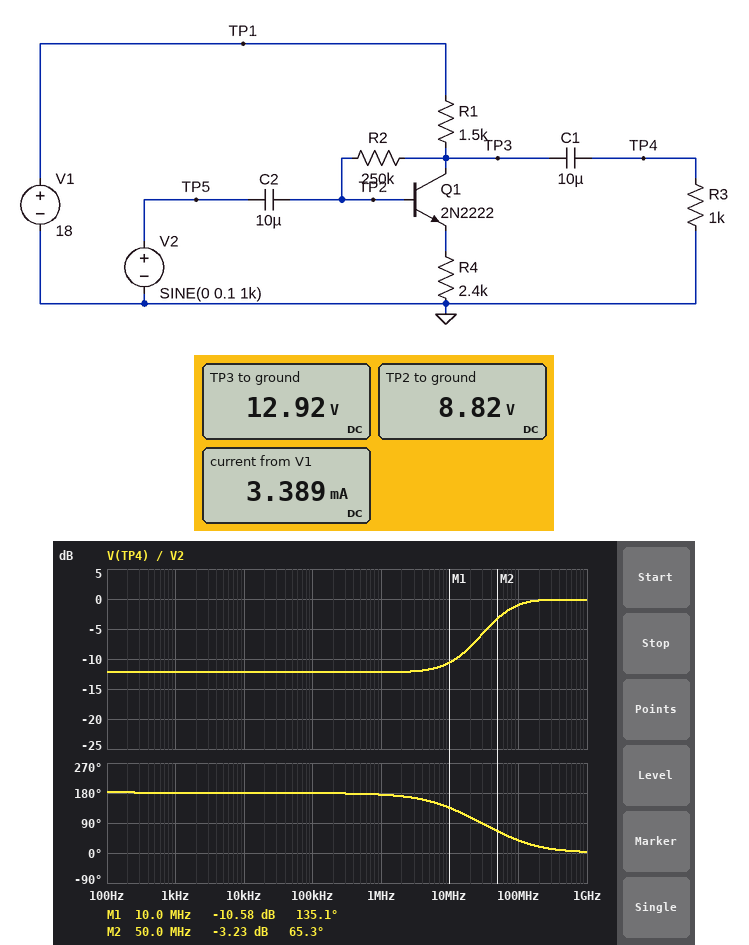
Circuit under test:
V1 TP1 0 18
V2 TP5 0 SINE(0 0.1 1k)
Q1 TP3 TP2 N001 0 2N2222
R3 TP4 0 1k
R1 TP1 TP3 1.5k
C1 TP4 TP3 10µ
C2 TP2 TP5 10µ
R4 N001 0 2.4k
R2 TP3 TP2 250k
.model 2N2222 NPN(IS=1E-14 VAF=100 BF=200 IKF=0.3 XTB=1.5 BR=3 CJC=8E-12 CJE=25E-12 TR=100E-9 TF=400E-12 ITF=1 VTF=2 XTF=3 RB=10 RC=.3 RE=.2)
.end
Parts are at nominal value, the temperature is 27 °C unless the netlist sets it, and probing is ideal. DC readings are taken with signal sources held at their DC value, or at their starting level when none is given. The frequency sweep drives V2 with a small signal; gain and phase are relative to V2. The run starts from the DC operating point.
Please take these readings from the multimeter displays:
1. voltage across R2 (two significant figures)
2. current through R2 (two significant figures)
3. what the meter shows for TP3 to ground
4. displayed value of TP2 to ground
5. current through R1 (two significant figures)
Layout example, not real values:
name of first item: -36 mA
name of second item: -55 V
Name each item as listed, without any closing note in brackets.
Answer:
voltage across R2: 4.1 V
current through R2: 16 µA
what the meter shows for TP3 to ground: 12.92 V
displayed value of TP2 to ground: 8.82 V
current through R1: 3.4 mA
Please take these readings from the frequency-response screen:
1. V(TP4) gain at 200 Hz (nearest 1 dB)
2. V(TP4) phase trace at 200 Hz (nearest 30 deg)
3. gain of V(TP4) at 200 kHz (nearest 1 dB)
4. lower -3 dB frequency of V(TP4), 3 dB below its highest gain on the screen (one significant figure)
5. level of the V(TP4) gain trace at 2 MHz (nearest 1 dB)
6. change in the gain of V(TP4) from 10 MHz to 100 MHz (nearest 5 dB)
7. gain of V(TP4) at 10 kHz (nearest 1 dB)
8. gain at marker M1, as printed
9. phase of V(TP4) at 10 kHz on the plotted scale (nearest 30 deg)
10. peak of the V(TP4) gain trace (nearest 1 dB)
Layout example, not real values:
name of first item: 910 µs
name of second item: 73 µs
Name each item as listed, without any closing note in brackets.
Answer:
V(TP4) gain at 200 Hz: -12 dB
V(TP4) phase trace at 200 Hz: 180 deg
gain of V(TP4) at 200 kHz: -12 dB
lower -3 dB frequency of V(TP4), 3 dB below its highest gain on the screen: 50 MHz
level of the V(TP4) gain trace at 2 MHz: -12 dB
change in the gain of V(TP4) from 10 MHz to 100 MHz: 10 dB
gain of V(TP4) at 10 kHz: -12 dB
gain at marker M1, as printed: -10.58 dB
phase of V(TP4) at 10 kHz on the plotted scale: 180 deg
peak of the V(TP4) gain trace: 0 dB
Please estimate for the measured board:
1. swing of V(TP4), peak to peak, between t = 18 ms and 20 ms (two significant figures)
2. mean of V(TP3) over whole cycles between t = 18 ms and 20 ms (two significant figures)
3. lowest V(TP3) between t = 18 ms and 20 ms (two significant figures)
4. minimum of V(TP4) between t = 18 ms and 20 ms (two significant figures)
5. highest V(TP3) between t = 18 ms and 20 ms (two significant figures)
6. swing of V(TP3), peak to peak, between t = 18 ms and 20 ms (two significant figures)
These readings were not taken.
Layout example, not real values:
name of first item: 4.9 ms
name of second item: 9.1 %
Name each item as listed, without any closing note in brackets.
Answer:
swing of V(TP4), peak to peak, between t = 18 ms and 20 ms: 49 mV
mean of V(TP3) over whole cycles between t = 18 ms and 20 ms: 13 V
lowest V(TP3) between t = 18 ms and 20 ms: 13 V
minimum of V(TP4) between t = 18 ms and 20 ms: -24 mV
highest V(TP3) between t = 18 ms and 20 ms: 13 V
swing of V(TP3), peak to peak, between t = 18 ms and 20 ms: 49 mV
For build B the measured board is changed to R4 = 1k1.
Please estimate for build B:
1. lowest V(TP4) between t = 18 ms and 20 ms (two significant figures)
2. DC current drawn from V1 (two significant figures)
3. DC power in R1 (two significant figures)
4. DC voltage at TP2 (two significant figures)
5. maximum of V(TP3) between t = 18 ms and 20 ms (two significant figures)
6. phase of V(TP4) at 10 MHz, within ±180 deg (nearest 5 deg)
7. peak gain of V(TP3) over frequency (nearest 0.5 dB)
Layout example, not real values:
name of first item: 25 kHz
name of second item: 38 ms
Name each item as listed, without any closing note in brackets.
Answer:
lowest V(TP4) between t = 18 ms and 20 ms: -53 mV
DC current drawn from V1: 4.6 mA
DC power in R1: 31 mW
DC voltage at TP2: 5.7 V
maximum of V(TP3) between t = 18 ms and 20 ms: 11 V
phase of V(TP4) at 10 MHz, within ±180 deg: 155 deg
peak gain of V(TP3) over frequency: 2.5 dB
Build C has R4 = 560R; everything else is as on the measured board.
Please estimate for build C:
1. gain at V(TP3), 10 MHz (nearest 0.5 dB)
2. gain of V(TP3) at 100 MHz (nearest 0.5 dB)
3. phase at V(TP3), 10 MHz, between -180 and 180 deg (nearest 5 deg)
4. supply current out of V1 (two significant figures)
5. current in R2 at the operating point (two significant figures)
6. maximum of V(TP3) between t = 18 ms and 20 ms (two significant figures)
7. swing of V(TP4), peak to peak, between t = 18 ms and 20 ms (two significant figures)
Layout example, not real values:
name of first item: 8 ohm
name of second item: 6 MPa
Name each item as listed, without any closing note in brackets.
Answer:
gain at V(TP3), 10 MHz: 0.5 dB
gain of V(TP3) at 100 MHz: 1.0 dB
phase at V(TP3), 10 MHz, between -180 and 180 deg: 160 deg
supply current out of V1: 5.3 mA
current in R2 at the operating point: 25 µA
maximum of V(TP3) between t = 18 ms and 20 ms: 10 V
swing of V(TP4), peak to peak, between t = 18 ms and 20 ms: 210 mV
